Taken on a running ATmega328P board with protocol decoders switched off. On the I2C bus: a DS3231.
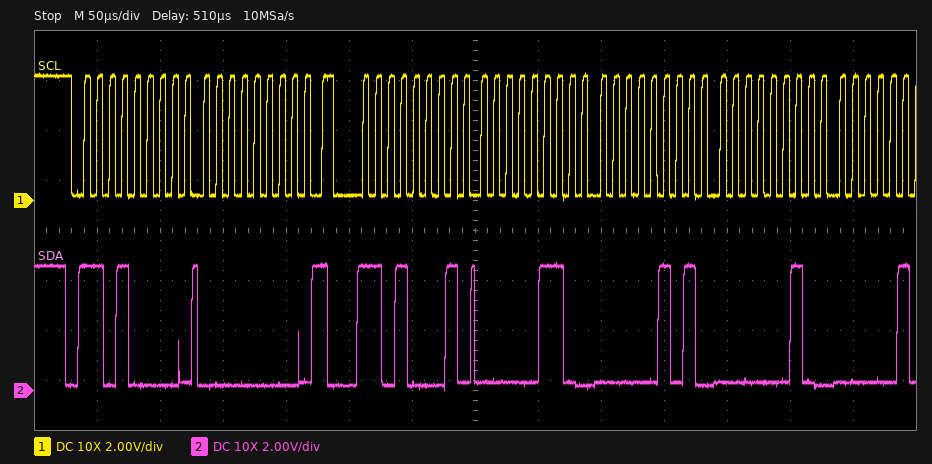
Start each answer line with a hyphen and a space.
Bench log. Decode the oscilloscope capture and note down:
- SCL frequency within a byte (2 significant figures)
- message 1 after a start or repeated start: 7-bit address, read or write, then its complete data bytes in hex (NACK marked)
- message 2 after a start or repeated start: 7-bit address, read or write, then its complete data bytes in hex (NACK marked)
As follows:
- 100 kHz
- 0x68 write: 00
- 0x68 read: 06 05 02
